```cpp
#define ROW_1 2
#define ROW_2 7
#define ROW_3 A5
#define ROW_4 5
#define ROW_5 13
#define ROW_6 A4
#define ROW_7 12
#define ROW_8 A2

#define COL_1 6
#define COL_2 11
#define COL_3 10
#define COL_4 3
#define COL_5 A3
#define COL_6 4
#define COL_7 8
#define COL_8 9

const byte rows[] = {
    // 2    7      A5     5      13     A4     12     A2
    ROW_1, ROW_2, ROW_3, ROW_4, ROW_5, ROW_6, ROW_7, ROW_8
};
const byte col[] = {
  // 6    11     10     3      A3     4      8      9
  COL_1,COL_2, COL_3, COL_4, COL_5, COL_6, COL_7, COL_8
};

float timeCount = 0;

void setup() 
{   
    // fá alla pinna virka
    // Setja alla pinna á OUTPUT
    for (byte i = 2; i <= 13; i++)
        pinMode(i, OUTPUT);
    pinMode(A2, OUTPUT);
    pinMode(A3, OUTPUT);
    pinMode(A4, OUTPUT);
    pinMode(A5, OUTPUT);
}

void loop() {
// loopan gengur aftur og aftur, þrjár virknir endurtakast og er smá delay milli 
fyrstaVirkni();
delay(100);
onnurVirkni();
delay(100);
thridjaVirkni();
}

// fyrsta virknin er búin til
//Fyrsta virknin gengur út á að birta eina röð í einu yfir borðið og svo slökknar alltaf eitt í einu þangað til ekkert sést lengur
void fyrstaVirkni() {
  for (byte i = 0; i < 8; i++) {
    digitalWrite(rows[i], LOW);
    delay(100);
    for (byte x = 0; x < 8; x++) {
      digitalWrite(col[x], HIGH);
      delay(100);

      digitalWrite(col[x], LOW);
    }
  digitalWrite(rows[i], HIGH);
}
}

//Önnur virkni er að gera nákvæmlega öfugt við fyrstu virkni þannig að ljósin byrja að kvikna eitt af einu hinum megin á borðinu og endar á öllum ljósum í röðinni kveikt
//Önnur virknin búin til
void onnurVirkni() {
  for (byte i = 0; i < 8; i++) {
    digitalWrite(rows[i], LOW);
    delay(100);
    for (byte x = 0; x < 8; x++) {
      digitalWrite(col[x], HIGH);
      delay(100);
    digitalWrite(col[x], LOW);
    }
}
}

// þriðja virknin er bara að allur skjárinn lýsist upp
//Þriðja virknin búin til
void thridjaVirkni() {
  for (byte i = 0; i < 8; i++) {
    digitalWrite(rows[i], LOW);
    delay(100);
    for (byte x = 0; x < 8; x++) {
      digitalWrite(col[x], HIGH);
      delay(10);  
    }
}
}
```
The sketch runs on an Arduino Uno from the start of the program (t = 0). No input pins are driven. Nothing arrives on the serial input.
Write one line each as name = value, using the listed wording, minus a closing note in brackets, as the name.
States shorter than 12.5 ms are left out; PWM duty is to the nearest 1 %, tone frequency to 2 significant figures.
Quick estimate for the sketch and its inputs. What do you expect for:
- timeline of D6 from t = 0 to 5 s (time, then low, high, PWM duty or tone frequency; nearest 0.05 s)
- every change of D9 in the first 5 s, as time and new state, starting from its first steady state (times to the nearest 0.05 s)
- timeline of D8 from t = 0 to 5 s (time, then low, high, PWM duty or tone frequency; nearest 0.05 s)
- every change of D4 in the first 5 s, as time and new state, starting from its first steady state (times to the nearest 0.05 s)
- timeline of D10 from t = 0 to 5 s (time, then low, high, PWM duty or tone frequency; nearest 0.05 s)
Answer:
timeline of D6 from t = 0 to 5 s = 0 s low; 0.1 s high; 0.2 s low; 1 s high; 1.1 s low; 1.9 s high; 2 s low; 2.8 s high; 2.9 s low; 3.7 s high; 3.8 s low; 4.6 s high; 4.7 s low
every change of D9 in the first 5 s, as time and new state, starting from its first steady state = 0 s low; 0.8 s high; 0.9 s low; 1.7 s high; 1.8 s low; 2.6 s high; 2.7 s low; 3.5 s high; 3.6 s low; 4.4 s high; 4.5 s low
timeline of D8 from t = 0 to 5 s = 0 s low; 0.7 s high; 0.8 s low; 1.6 s high; 1.7 s low; 2.5 s high; 2.6 s low; 3.4 s high; 3.5 s low; 4.3 s high; 4.4 s low
every change of D4 in the first 5 s, as time and new state, starting from its first steady state = 0 s low; 0.6 s high; 0.7 s low; 1.5 s high; 1.6 s low; 2.4 s high; 2.5 s low; 3.3 s high; 3.4 s low; 4.2 s high; 4.3 s low
timeline of D10 from t = 0 to 5 s = 0 s low; 0.3 s high; 0.4 s low; 1.2 s high; 1.3 s low; 2.1 s high; 2.2 s low; 3 s high; 3.1 s low; 3.9 s high; 4 s low; 4.8 s high; 4.9 s low
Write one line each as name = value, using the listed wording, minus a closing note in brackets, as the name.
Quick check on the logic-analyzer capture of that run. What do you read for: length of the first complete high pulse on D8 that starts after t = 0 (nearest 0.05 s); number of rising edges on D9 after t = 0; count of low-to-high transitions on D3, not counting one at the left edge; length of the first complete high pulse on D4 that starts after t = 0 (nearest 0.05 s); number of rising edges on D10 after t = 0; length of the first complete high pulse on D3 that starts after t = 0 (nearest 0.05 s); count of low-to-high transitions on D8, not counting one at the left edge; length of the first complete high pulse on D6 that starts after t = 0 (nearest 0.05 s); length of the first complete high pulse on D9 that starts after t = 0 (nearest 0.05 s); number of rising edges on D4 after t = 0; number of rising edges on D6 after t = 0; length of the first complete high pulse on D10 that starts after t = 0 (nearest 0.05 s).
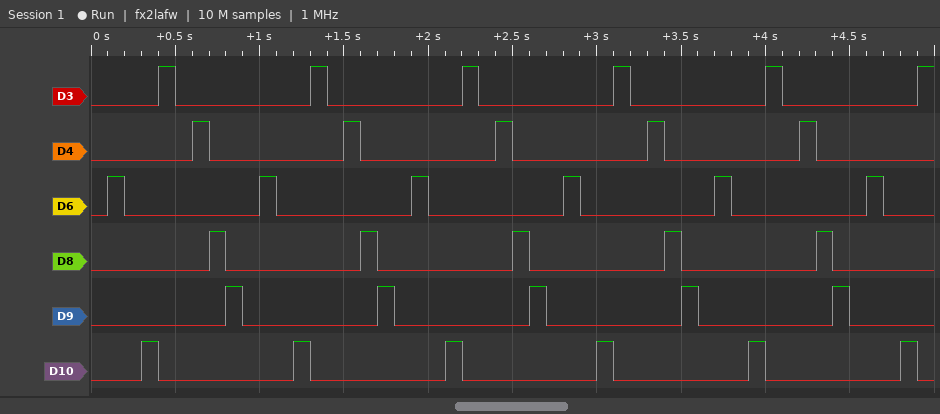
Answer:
length of the first complete high pulse on D8 that starts after t = 0 = 0.10 s
number of rising edges on D9 after t = 0 = 5
count of low-to-high transitions on D3, not counting one at the left edge = 6
length of the first complete high pulse on D4 that starts after t = 0 = 0.10 s
number of rising edges on D10 after t = 0 = 6
length of the first complete high pulse on D3 that starts after t = 0 = 0.10 s
count of low-to-high transitions on D8, not counting one at the left edge = 5
length of the first complete high pulse on D6 that starts after t = 0 = 0.10 s
length of the first complete high pulse on D9 that starts after t = 0 = 0.10 s
number of rising edges on D4 after t = 0 = 5
number of rising edges on D6 after t = 0 = 6
length of the first complete high pulse on D10 that starts after t = 0 = 0.10 s
